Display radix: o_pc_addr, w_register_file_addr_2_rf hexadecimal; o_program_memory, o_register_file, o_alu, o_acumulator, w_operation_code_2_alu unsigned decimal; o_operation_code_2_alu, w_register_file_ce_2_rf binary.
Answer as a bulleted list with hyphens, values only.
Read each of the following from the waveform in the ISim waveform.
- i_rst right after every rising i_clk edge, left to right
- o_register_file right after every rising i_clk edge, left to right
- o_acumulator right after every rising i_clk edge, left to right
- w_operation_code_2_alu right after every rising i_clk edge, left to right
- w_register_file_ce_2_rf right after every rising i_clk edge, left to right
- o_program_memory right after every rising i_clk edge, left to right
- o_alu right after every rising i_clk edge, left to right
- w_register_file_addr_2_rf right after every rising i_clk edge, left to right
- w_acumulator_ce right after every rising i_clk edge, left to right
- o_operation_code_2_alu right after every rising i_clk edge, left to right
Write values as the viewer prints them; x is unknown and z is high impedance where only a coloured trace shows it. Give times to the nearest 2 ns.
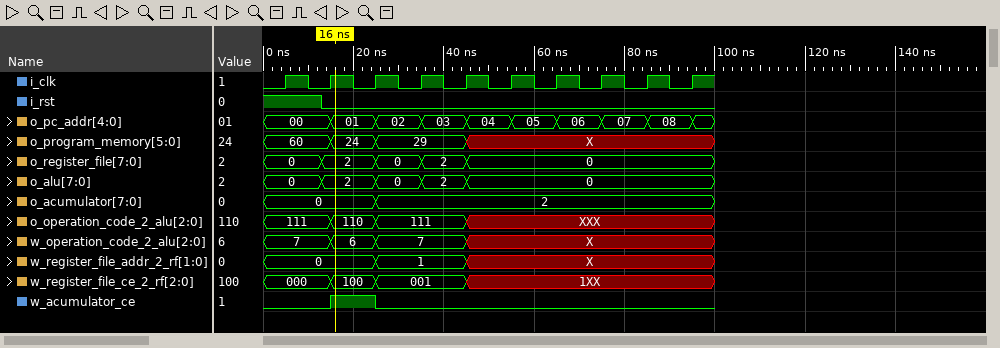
- 1 0 0 0 0 0 0 0 0 0
- 0, 2, 0, 2, 0, 0, 0, 0, 0, 0
- 0, 0, 2, 2, 2, 2, 2, 2, 2, 2
- 7, 6, 7, 7, X, X, X, X, X, X
- 000, 100, 001, 001, 1XX, 1XX, 1XX, 1XX, 1XX, 1XX
- 60, 24, 29, 29, X, X, X, X, X, X
- 0, 2, 0, 2, 0, 0, 0, 0, 0, 0
- 0, 0, 1, 1, X, X, X, X, X, X
- 0 1 0 0 0 0 0 0 0 0
- 111, 110, 111, 111, XXX, XXX, XXX, XXX, XXX, XXX
